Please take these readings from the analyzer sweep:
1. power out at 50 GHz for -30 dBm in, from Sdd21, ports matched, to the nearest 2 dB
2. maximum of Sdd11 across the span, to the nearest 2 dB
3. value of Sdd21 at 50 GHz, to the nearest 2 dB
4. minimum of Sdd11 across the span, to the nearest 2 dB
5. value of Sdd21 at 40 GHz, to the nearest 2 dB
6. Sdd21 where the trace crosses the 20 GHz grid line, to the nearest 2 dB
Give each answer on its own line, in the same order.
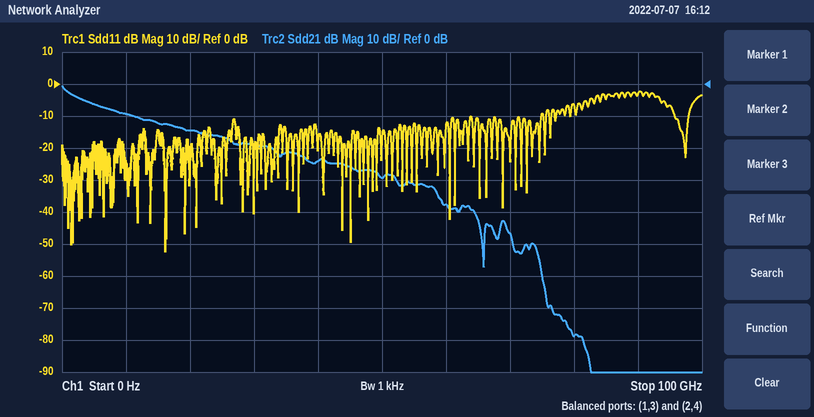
-60 dBm
-2 dB
-30 dB
-52 dB
-24 dB
-14 dB
